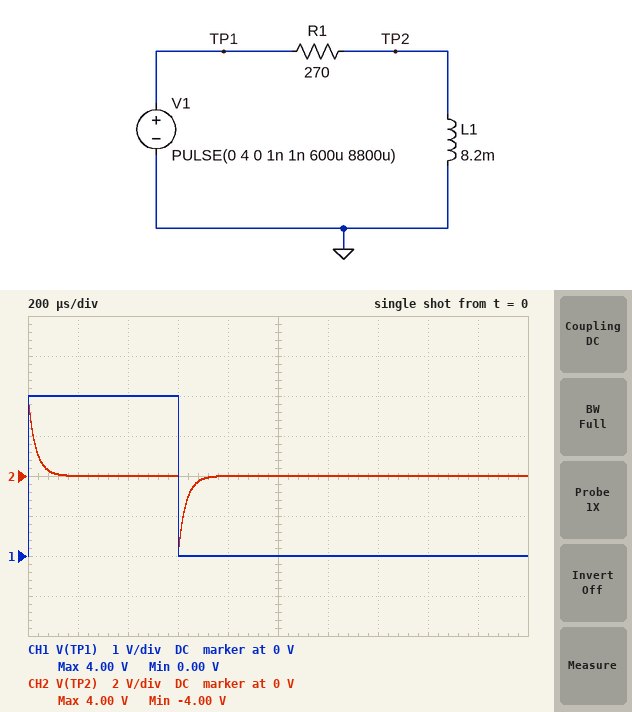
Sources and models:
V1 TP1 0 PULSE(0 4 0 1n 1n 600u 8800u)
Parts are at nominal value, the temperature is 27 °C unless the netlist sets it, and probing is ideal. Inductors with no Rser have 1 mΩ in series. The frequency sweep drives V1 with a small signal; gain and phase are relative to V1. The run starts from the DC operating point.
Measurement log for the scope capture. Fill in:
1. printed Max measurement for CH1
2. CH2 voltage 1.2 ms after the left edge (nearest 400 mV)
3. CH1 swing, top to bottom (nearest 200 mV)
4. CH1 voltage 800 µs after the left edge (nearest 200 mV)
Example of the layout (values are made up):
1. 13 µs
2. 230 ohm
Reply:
1. 4.00 V
2. 0 V
3. 4.0 V
4. 0 V
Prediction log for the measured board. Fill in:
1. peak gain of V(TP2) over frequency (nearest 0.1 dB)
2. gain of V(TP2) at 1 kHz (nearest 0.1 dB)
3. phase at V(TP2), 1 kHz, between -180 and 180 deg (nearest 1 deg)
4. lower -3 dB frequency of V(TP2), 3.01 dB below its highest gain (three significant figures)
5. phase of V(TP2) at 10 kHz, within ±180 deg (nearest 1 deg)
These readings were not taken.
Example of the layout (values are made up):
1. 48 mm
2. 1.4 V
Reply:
1. 0 dB
2. -14.5 dB
3. 79 deg
4. 5.24 kHz
5. 28 deg
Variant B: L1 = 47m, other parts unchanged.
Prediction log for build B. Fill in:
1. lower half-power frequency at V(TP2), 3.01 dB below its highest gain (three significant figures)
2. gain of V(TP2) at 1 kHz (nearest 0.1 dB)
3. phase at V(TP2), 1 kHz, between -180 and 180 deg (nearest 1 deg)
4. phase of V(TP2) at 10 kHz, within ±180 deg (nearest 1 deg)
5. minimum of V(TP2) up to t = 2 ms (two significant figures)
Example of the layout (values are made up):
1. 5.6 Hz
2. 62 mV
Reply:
1. 914 Hz
2. -2.6 dB
3. 42 deg
4. 5 deg
5. -3.9 V
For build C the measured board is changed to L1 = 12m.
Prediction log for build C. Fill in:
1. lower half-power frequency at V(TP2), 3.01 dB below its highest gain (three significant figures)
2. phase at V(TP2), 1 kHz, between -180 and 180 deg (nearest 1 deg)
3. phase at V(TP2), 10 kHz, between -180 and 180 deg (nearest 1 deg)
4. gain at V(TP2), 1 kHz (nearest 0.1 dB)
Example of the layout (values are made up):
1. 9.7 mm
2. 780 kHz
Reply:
1. 3.58 kHz
2. 74 deg
3. 20 deg
4. -11.4 dB
